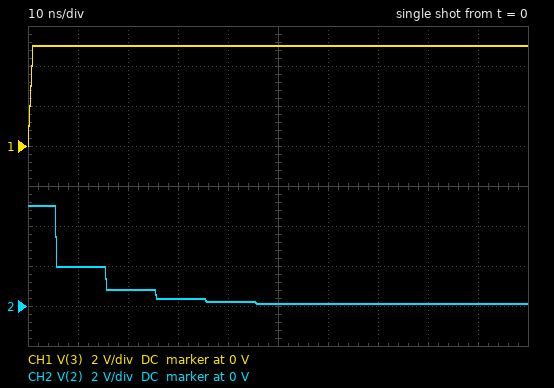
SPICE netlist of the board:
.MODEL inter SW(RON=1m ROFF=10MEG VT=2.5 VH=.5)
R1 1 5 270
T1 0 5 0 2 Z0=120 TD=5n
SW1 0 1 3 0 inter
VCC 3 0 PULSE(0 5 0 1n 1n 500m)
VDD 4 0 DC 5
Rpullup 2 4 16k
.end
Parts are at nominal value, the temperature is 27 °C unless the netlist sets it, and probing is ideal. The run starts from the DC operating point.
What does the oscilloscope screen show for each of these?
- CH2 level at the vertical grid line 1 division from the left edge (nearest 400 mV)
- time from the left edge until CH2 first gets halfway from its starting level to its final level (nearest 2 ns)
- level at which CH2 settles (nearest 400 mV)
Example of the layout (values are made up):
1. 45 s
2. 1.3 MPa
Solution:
1. 2.0 V
2. 6 ns
3. 0 V
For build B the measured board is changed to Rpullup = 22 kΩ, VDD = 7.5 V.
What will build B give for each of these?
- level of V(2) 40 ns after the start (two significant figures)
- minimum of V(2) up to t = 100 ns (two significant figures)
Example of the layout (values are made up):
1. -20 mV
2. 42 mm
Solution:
1. 250 mV
2. 91 mV
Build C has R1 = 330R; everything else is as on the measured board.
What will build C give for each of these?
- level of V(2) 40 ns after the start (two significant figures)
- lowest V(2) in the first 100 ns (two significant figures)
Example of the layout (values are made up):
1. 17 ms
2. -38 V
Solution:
1. 320 mV
2. 100 mV
